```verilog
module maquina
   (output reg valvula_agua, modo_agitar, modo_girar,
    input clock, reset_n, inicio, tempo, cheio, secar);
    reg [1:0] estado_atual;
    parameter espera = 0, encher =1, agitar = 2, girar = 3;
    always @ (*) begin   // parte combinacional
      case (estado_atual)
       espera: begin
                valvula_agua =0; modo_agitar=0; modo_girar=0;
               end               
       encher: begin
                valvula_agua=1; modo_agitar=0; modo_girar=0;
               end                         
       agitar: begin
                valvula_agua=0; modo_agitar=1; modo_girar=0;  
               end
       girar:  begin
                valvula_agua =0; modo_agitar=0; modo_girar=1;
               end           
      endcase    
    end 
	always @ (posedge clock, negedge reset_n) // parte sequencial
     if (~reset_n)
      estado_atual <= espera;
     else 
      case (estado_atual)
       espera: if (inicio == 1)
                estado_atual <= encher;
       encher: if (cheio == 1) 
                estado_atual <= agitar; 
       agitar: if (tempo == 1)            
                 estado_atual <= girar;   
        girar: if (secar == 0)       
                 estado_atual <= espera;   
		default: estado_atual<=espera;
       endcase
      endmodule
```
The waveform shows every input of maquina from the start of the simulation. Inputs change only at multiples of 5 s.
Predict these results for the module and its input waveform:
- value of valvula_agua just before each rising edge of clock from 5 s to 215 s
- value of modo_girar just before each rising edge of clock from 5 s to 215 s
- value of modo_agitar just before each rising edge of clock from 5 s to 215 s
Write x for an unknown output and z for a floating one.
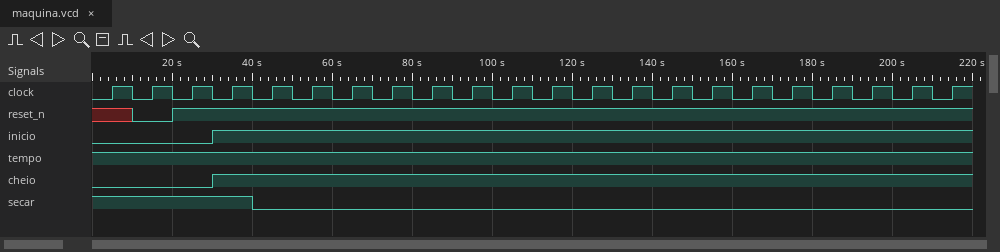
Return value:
x 0 0 0 1 0 0 0 1 0 0 0 1 0 0 0 1 0 0 0 1 0
x 0 0 0 0 0 1 0 0 0 1 0 0 0 1 0 0 0 1 0 0 0
x 0 0 0 0 1 0 0 0 1 0 0 0 1 0 0 0 1 0 0 0 1
